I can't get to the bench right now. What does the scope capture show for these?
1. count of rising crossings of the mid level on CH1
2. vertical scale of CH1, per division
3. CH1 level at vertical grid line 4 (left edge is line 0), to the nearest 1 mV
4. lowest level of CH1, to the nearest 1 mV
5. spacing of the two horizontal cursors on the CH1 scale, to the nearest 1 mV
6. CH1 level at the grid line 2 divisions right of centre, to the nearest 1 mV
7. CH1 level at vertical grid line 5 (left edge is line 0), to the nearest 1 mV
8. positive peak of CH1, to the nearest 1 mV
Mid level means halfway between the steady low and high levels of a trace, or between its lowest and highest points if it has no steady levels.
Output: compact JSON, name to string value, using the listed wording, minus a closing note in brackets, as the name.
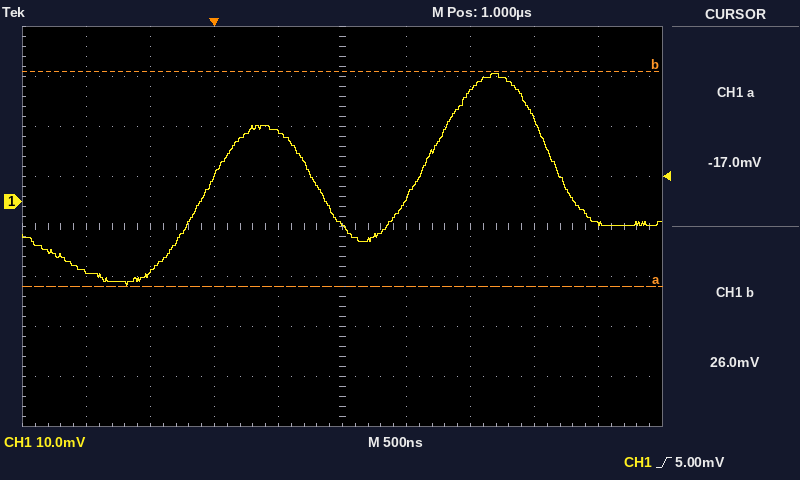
{"count of rising crossings of the mid level on CH1": "2", "vertical scale of CH1, per division": "10 mV", "CH1 level at vertical grid line 4 (left edge is line 0), to the nearest 1 mV": "14 mV", "lowest level of CH1, to the nearest 1 mV": "-17 mV", "spacing of the two horizontal cursors on the CH1 scale, to the nearest 1 mV": "43 mV", "CH1 level at the grid line 2 divisions right of centre, to the nearest 1 mV": "22 mV", "CH1 level at vertical grid line 5 (left edge is line 0), to the nearest 1 mV": "-5 mV", "positive peak of CH1, to the nearest 1 mV": "26 mV"}
